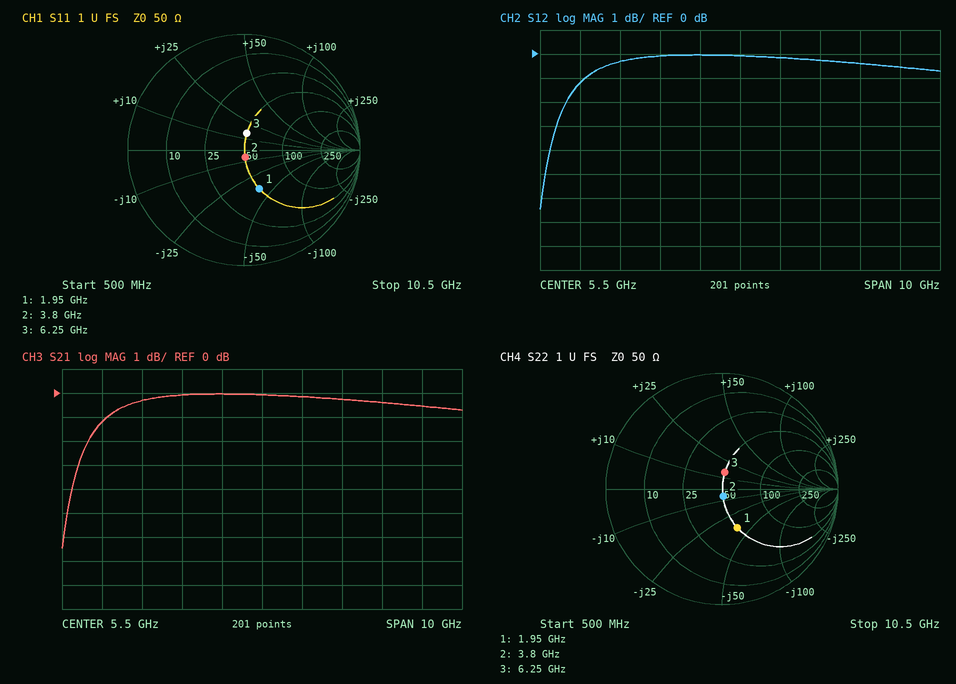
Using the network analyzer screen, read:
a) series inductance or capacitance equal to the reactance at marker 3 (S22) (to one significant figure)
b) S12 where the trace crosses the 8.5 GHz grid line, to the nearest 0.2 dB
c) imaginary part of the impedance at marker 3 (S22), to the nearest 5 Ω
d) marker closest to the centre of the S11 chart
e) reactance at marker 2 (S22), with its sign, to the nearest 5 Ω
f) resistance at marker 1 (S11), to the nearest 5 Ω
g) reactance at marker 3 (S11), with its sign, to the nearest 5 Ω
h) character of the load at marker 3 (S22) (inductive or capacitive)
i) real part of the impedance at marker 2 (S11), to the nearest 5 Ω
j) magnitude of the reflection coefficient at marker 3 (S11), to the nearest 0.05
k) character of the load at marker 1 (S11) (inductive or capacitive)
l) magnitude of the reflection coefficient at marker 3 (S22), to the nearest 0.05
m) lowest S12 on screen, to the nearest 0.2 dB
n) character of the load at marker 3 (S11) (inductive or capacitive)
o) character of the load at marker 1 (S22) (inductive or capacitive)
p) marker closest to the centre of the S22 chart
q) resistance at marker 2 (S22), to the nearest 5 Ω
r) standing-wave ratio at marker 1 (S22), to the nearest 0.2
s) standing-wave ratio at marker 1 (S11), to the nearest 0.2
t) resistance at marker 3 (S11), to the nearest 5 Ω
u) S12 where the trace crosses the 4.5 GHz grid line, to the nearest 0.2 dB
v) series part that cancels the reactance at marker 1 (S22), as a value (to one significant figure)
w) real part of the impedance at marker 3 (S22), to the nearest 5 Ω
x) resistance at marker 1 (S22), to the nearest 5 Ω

400 pH
-0.4 dB
+15 Ω
marker 2
-5 Ω
50 Ω
+15 Ω
inductive
50 Ω
0.15
capacitive
0.15
-6.4 dB
inductive
capacitive
marker 2
50 Ω
2.2
2.2
50 Ω
0.0 dB
3 nH
50 Ω
50 Ω
